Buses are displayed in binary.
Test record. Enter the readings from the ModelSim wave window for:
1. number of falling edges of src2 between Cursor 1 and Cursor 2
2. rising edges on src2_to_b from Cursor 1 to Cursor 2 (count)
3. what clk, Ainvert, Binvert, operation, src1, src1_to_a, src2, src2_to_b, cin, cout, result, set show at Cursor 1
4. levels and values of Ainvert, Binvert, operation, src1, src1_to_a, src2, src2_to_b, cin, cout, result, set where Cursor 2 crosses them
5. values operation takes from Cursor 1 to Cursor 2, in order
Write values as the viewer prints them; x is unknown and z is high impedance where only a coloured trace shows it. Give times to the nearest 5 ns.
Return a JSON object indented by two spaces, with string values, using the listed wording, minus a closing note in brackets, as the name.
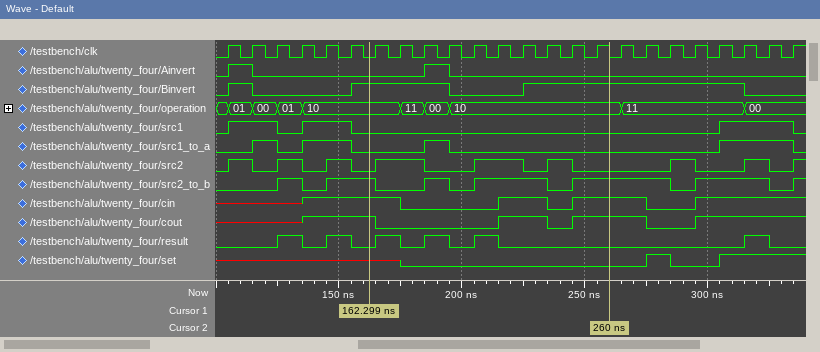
{
  "number of falling edges of src2 between Cursor 1 and Cursor 2": "3",
  "rising edges on src2_to_b from Cursor 1 to Cursor 2": "3",
  "what clk, Ainvert, Binvert, operation, src1, src1_to_a, src2, src2_to_b, cin, cout, result, set show at Cursor 1": "clk=0, Ainvert=0, Binvert=1, operation=10, src1=0, src1_to_a=0, src2=0, src2_to_b=1, cin=1, cout=1, result=0, set=x",
  "levels and values of Ainvert, Binvert, operation, src1, src1_to_a, src2, src2_to_b, cin, cout, result, set where Cursor 2 crosses them": "Ainvert=0, Binvert=1, operation=10, src1=0, src1_to_a=0, src2=0, src2_to_b=1, cin=1, cout=1, result=0, set=0",
  "values operation takes from Cursor 1 to Cursor 2, in order": "10, 11, 00, 10"
}
